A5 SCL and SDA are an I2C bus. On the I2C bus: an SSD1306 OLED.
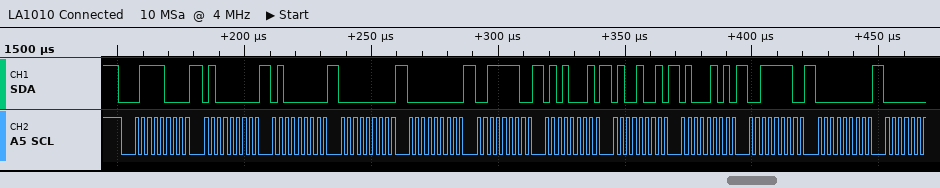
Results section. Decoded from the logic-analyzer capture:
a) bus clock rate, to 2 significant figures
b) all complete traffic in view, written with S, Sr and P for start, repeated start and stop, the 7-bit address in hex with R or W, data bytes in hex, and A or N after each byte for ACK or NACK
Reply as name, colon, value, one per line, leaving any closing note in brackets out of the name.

bus clock rate, to 2 significant figures: 400 kHz
all complete traffic in view, written with S, Sr and P for start, repeated start and stop, the 7-bit address in hex with R or W, data bytes in hex, and A or N after each byte for ACK or NACK: S 3CW A 40 A 40 A 00 A 00 A 3E A 51 A 49 A 45 A 3E A 00 A
